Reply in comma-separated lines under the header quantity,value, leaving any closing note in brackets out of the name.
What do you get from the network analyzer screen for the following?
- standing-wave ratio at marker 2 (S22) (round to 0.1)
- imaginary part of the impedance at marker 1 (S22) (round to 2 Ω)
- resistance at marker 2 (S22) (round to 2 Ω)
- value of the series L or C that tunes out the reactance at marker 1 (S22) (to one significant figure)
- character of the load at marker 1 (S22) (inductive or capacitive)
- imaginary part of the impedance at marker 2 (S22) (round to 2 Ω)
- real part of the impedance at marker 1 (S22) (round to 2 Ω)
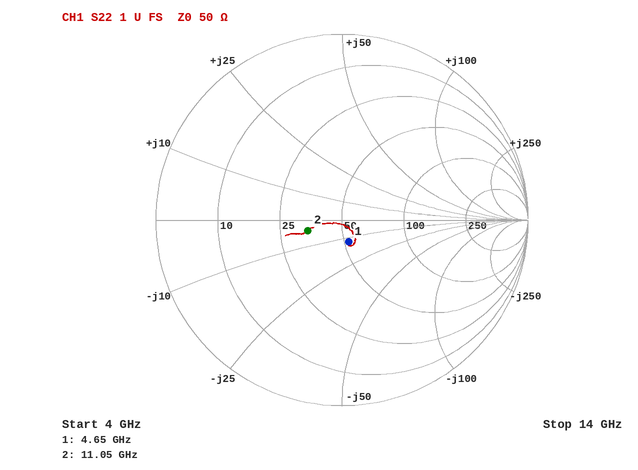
quantity,value
standing-wave ratio at marker 2 (S22),1.5
imaginary part of the impedance at marker 1 (S22),-12 Ω
resistance at marker 2 (S22),34 Ω
value of the series L or C that tunes out the reactance at marker 1 (S22),400 pH
character of the load at marker 1 (S22),capacitive
imaginary part of the impedance at marker 2 (S22),-4 Ω
real part of the impedance at marker 1 (S22),52 Ω
